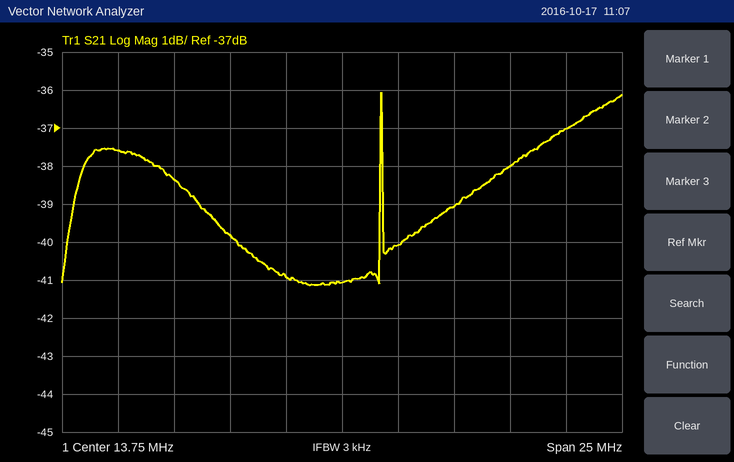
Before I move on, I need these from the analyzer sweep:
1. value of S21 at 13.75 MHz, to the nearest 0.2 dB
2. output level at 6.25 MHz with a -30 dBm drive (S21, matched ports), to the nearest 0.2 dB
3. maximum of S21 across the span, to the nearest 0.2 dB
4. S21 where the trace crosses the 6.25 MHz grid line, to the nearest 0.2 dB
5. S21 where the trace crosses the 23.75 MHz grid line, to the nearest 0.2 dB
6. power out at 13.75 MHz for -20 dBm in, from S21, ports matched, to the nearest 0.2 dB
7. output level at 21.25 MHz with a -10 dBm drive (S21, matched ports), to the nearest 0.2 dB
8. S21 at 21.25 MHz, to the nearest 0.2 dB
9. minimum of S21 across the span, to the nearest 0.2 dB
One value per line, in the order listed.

-41.0 dB
-68.4 dBm
-36.0 dB
-38.4 dB
-37.0 dB
-61.0 dBm
-48.0 dBm
-38.0 dB
-41.2 dB
